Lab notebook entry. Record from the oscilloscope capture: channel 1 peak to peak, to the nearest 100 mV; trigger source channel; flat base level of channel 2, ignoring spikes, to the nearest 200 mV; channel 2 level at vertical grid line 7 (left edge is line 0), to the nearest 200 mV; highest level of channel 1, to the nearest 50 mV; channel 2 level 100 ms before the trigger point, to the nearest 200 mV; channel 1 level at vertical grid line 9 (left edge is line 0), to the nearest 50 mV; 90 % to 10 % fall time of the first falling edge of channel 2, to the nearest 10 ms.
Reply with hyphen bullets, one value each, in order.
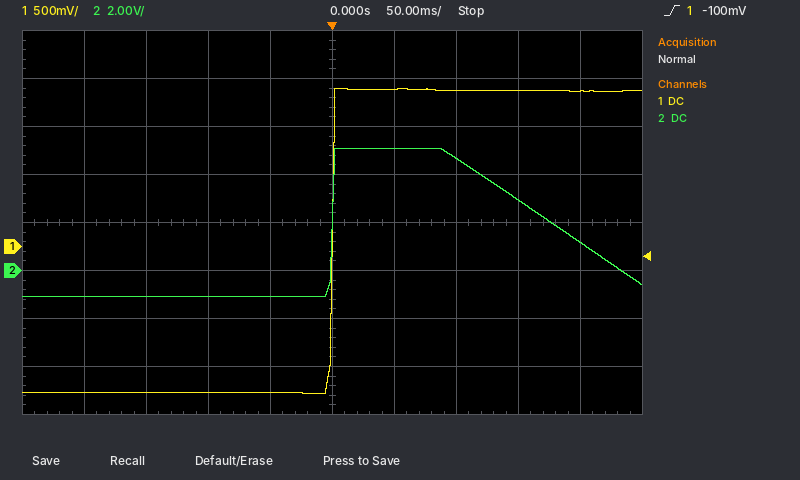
- 3.20 V
- channel 1
- -1.0 V
- 4.6 V
- 1.65 V
- -1.0 V
- 1.60 V
- 140 ms
